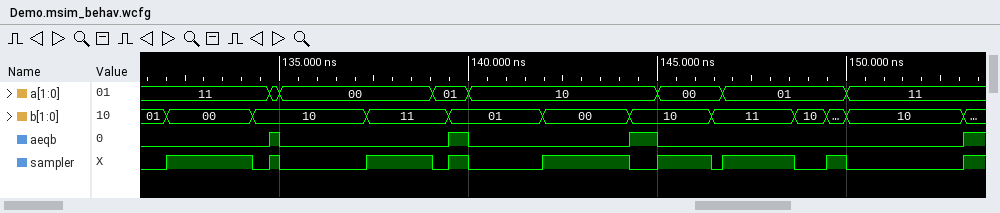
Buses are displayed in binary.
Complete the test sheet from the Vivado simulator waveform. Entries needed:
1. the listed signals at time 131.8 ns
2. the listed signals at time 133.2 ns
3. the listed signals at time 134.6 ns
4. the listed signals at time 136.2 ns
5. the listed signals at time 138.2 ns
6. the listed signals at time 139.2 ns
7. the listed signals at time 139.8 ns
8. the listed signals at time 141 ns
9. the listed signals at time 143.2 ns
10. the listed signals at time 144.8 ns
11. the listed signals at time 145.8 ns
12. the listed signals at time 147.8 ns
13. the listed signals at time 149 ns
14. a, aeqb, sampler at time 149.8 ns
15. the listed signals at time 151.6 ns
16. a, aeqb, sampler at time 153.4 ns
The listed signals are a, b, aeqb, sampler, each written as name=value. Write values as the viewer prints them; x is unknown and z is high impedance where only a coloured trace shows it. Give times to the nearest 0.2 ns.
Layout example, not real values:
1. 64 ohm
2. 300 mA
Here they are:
1. a=11, b=01, aeqb=0, sampler=0
2. a=11, b=00, aeqb=0, sampler=1
3. a=11, b=10, aeqb=0, sampler=0
4. a=00, b=10, aeqb=0, sampler=0
5. a=00, b=11, aeqb=0, sampler=1
6. a=01, b=11, aeqb=0, sampler=0
7. a=01, b=01, aeqb=1, sampler=1
8. a=10, b=01, aeqb=0, sampler=0
9. a=10, b=00, aeqb=0, sampler=1
10. a=10, b=10, aeqb=1, sampler=0
11. a=00, b=10, aeqb=0, sampler=1
12. a=01, b=11, aeqb=0, sampler=1
13. a=01, b=10, aeqb=0, sampler=0
14. a=01, aeqb=0, sampler=1
15. a=11, b=10, aeqb=0, sampler=0
16. a=11, aeqb=1, sampler=1
